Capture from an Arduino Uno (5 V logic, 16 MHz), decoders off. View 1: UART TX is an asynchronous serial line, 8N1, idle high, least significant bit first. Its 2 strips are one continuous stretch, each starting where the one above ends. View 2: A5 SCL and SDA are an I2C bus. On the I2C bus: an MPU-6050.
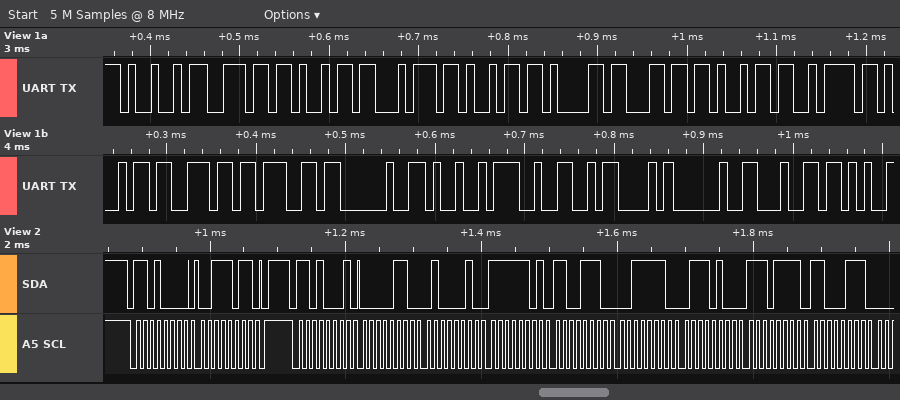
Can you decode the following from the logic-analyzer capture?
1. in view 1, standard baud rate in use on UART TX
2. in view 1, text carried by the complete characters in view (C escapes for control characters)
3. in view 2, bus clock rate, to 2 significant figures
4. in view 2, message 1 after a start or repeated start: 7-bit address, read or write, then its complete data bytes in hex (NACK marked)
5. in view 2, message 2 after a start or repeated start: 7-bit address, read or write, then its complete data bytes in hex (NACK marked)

115200 baud
"Initializing I2C d"
100 kHz
0x68 write: 3B
0x68 read: 06 42 FD CE 3E 74 EF C7
